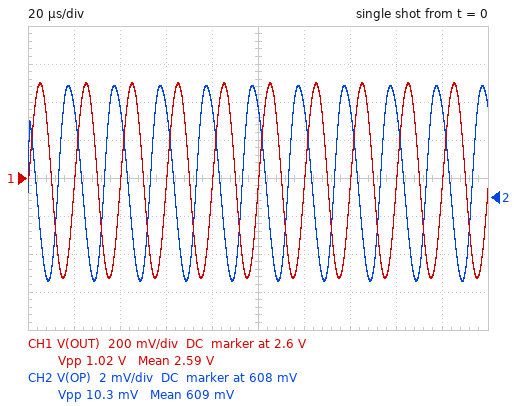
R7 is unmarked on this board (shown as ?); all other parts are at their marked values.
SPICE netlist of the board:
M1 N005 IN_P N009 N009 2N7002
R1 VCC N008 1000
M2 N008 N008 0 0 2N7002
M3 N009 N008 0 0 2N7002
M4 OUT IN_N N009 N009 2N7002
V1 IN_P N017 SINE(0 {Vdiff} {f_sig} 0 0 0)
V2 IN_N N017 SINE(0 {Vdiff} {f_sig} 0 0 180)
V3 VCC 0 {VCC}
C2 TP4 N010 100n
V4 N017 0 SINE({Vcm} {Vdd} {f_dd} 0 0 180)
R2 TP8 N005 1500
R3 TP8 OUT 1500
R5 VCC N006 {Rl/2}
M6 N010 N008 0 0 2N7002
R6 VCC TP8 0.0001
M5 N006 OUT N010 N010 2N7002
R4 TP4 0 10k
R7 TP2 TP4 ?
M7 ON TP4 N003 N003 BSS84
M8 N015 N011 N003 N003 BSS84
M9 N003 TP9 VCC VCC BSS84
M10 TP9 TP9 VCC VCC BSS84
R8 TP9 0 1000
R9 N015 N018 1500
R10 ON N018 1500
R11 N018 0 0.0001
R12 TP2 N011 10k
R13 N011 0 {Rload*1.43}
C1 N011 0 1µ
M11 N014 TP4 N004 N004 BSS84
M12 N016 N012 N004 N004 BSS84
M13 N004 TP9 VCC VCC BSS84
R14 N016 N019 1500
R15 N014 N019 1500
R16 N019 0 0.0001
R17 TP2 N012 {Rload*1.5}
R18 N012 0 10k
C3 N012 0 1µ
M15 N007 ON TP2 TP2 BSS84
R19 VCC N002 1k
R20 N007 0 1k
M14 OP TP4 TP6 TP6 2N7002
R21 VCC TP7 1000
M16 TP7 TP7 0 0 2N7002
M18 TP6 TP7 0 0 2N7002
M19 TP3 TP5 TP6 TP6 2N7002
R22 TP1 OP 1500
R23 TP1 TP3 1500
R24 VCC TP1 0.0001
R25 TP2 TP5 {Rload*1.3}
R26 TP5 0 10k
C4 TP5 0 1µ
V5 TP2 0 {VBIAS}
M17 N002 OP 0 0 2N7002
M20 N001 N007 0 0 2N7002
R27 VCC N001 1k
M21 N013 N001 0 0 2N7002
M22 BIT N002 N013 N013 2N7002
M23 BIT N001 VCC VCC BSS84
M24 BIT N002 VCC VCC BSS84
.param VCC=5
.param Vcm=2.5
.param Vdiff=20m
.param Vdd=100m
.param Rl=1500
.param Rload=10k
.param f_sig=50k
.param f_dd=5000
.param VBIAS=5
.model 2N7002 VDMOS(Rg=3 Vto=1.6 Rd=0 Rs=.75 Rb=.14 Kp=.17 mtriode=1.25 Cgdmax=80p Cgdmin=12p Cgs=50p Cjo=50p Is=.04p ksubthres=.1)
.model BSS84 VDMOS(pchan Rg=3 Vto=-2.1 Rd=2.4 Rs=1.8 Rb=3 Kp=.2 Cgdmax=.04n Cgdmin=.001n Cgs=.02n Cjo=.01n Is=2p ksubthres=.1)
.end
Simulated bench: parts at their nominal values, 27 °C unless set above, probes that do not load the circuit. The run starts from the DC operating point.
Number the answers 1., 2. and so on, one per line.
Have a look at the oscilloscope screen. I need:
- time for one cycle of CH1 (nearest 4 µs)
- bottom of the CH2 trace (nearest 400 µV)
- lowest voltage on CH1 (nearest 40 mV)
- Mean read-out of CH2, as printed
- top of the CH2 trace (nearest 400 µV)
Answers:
1. 20 µs
2. 603.6 mV
3. 2.08 V
4. 609 mV
5. 614.0 mV
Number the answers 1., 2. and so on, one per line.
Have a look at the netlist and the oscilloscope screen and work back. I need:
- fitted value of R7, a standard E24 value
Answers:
1. 3.6 kΩ
